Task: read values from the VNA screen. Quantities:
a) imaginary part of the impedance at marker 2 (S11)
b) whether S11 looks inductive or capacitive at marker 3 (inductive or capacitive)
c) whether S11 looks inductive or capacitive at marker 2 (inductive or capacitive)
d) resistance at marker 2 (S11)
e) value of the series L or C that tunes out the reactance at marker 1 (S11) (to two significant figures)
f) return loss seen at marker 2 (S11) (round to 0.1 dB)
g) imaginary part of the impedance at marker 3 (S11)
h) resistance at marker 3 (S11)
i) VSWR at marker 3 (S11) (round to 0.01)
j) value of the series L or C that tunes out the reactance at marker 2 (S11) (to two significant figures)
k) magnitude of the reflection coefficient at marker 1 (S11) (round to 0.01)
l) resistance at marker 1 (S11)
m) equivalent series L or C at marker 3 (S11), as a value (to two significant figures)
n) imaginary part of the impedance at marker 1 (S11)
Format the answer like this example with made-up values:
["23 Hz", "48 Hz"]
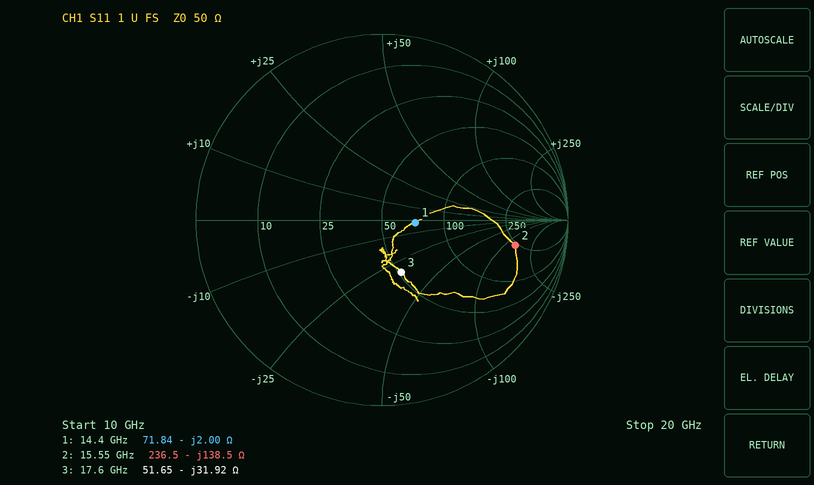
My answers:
["-138.5 Ω", "capacitive", "capacitive", "236.5 Ω", "22 pH", "2.7 dB", "-31.92 Ω", "51.65 Ω", "1.86", "1.4 nH", "0.18", "71.84 Ω", "280 fF", "-2.00 Ω"]
